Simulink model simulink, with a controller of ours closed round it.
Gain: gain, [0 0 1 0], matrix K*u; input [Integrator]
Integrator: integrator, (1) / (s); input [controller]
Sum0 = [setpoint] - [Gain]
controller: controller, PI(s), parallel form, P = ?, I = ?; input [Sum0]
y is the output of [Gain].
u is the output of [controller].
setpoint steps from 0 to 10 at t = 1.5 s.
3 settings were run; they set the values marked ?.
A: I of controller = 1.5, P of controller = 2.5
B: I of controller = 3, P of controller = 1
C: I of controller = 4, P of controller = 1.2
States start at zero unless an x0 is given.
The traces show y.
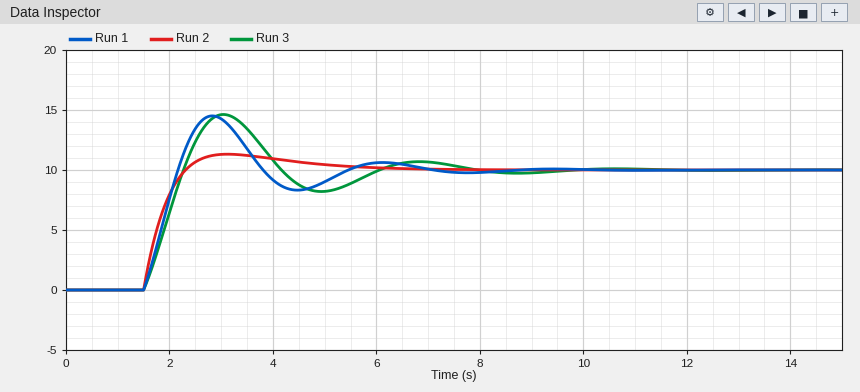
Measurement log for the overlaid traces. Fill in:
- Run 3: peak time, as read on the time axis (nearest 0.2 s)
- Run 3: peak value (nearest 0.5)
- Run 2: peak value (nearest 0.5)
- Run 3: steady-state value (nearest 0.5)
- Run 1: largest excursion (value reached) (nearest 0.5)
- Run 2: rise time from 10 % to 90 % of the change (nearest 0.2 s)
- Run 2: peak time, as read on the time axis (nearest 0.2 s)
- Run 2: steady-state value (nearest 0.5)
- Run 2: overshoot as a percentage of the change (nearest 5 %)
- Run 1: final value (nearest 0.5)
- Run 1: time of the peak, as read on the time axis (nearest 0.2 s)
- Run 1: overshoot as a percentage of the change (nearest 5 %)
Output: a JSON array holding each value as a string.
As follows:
["3.0 s", "14.5", "11.5", "10.0", "14.5", "0.6 s", "3.2 s", "10.0", "15 %", "10.0", "2.8 s", "45 %"]
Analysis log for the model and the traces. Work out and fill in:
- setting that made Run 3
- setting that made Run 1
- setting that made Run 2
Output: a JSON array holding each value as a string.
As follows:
["B", "C", "A"]
